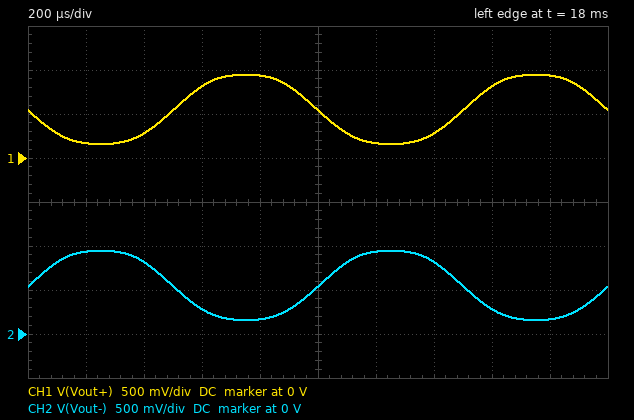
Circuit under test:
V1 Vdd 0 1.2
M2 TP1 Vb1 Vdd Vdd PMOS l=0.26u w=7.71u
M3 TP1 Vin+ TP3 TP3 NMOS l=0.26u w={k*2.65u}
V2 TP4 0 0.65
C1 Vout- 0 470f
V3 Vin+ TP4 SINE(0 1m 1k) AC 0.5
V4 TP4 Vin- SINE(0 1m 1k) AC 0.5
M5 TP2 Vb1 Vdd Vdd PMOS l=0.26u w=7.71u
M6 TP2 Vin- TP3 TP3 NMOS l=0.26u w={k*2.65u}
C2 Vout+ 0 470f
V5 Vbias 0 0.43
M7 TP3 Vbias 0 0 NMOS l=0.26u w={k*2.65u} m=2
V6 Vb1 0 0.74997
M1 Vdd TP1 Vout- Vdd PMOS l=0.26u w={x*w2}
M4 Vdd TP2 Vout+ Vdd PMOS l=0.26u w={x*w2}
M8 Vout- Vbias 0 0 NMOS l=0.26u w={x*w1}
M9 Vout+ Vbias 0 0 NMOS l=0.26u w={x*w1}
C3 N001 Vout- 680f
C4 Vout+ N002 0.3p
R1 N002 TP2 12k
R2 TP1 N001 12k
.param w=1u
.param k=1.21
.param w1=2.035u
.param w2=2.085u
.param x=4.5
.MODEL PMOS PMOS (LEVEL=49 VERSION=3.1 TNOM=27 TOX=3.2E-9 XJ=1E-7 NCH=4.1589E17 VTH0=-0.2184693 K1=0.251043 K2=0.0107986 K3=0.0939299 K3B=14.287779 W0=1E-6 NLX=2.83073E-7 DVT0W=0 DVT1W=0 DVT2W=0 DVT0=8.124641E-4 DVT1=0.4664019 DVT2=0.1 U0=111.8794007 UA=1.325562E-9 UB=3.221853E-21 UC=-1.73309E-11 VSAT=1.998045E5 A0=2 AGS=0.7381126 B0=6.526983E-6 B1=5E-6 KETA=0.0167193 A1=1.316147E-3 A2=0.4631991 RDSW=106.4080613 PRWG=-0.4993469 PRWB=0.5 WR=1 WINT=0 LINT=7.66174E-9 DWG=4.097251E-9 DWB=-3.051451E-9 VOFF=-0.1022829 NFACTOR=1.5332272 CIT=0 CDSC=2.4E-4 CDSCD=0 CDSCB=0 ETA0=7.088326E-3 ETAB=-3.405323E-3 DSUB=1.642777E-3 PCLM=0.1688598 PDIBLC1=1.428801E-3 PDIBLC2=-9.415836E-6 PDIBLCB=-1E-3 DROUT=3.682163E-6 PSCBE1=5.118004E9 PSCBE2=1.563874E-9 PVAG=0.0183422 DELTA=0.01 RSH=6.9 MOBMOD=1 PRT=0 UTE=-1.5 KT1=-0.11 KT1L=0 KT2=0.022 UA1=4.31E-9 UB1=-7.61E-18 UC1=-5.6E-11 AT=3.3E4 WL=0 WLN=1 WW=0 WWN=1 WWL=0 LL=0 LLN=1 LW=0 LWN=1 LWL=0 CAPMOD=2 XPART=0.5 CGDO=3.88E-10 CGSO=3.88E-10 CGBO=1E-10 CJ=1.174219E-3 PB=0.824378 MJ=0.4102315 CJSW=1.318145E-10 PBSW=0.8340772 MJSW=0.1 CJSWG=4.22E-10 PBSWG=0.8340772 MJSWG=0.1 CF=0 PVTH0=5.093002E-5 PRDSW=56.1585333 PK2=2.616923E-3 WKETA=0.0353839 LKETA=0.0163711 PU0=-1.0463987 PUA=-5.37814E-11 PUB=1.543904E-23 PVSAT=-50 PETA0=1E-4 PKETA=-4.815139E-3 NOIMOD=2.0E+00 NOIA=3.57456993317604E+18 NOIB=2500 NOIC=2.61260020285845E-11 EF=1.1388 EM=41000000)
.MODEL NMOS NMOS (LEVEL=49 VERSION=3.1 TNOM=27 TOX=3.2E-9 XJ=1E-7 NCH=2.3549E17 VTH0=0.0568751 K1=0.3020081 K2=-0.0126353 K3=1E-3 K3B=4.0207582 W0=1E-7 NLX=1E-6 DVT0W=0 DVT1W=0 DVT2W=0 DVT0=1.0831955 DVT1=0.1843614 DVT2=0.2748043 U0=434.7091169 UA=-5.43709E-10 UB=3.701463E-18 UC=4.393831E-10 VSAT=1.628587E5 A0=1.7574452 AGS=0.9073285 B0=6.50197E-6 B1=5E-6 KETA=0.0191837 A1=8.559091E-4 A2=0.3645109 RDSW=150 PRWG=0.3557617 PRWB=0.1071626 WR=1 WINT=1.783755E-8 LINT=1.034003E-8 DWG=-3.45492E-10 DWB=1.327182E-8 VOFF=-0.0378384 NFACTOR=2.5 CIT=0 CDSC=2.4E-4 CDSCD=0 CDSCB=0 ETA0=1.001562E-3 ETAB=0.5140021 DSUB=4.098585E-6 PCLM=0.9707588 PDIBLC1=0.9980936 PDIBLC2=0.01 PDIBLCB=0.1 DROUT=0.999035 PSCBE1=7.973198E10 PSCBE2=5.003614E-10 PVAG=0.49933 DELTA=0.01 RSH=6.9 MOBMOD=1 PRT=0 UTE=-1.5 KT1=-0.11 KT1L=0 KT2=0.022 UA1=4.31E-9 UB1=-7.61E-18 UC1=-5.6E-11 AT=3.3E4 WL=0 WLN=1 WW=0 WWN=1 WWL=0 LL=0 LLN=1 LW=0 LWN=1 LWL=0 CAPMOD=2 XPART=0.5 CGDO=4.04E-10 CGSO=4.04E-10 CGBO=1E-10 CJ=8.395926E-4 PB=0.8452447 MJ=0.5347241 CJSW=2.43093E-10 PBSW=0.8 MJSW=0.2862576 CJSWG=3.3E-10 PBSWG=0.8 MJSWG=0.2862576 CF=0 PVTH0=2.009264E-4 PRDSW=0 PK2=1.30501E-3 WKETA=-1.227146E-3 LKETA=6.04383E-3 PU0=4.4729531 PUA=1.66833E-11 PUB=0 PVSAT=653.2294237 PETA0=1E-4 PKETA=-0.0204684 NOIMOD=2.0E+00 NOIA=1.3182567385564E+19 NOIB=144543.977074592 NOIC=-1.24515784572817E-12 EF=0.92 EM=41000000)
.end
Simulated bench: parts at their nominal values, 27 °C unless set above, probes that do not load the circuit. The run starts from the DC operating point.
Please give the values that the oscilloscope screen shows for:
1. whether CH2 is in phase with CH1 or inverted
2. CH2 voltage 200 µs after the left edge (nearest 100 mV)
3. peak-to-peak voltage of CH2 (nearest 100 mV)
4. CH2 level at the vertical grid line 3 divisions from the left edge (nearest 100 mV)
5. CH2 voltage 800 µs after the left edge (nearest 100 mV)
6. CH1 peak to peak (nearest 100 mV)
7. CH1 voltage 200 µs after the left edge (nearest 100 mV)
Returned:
inverted
900 mV
800 mV
300 mV
200 mV
800 mV
200 mV
